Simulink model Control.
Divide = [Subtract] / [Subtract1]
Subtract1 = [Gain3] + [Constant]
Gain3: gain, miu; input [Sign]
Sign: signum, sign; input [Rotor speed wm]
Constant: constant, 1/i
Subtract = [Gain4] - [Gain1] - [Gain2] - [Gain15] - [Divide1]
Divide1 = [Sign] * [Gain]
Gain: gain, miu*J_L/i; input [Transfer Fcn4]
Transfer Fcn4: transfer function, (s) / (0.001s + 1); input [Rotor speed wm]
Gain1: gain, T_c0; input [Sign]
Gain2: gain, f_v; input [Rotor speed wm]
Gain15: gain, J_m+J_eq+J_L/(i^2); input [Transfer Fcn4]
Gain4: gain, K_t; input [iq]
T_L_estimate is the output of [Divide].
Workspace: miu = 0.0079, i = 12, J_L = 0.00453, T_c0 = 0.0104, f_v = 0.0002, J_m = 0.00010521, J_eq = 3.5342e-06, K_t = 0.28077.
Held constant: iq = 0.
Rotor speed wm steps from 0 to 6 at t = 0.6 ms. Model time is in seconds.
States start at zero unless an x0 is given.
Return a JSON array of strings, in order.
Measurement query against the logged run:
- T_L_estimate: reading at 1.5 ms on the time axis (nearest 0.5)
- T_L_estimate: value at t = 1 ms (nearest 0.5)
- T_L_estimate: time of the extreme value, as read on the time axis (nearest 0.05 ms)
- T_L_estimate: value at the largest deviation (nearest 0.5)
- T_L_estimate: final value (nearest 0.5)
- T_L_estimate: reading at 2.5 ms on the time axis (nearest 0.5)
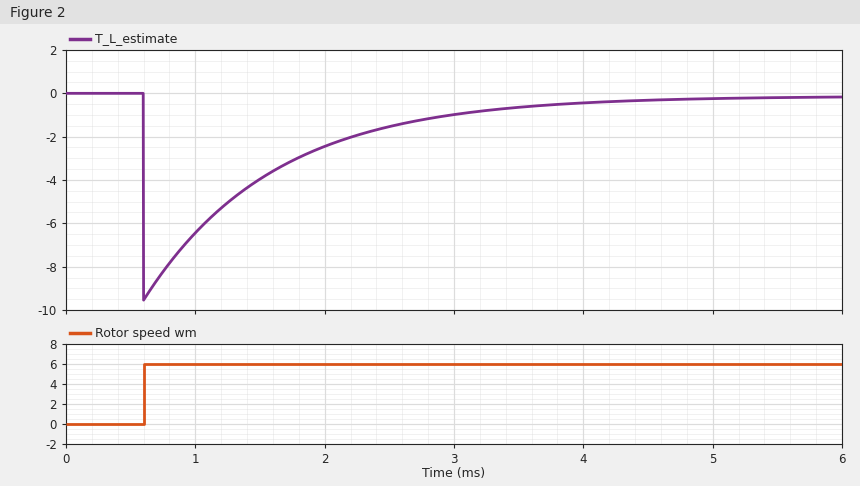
["-4.0", "-6.5", "0.60 ms", "-9.5", "0.0", "-1.5"]
